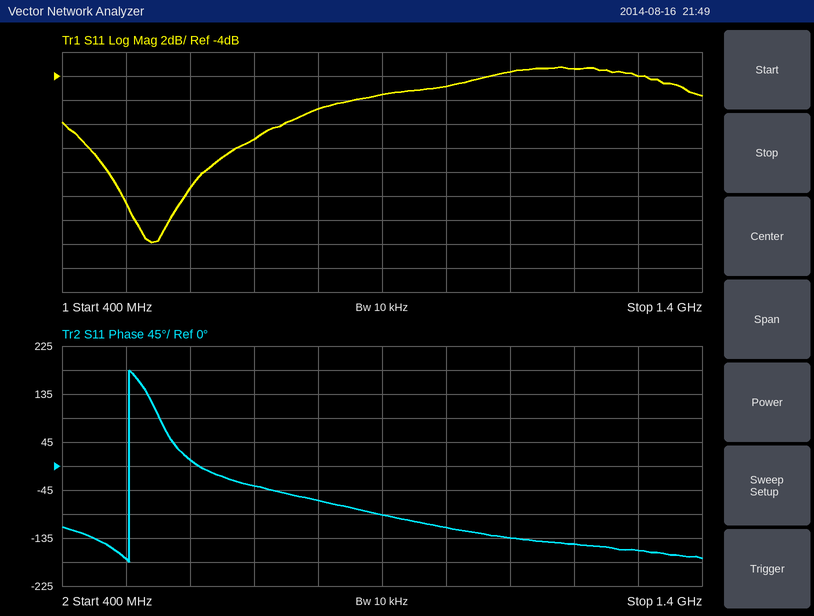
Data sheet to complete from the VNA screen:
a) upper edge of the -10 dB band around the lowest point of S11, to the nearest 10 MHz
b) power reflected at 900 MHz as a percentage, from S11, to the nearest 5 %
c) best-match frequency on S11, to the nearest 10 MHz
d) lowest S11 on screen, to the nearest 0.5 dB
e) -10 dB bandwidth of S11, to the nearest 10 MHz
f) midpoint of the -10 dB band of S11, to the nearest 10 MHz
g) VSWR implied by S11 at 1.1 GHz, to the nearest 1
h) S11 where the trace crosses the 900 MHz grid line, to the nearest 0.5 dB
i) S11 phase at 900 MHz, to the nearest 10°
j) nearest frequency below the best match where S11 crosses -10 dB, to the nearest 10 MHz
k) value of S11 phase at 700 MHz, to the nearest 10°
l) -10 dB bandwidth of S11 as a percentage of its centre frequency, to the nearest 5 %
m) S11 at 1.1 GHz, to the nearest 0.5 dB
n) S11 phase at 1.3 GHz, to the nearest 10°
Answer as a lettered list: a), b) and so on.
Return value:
a) 670 MHz
b) 30 %
c) 540 MHz
d) -18.0 dB
e) 230 MHz
f) 560 MHz
g) 5
h) -5.5 dB
i) -90°
j) 440 MHz
k) -40°
l) 40 %
m) -3.5 dB
n) -160°
